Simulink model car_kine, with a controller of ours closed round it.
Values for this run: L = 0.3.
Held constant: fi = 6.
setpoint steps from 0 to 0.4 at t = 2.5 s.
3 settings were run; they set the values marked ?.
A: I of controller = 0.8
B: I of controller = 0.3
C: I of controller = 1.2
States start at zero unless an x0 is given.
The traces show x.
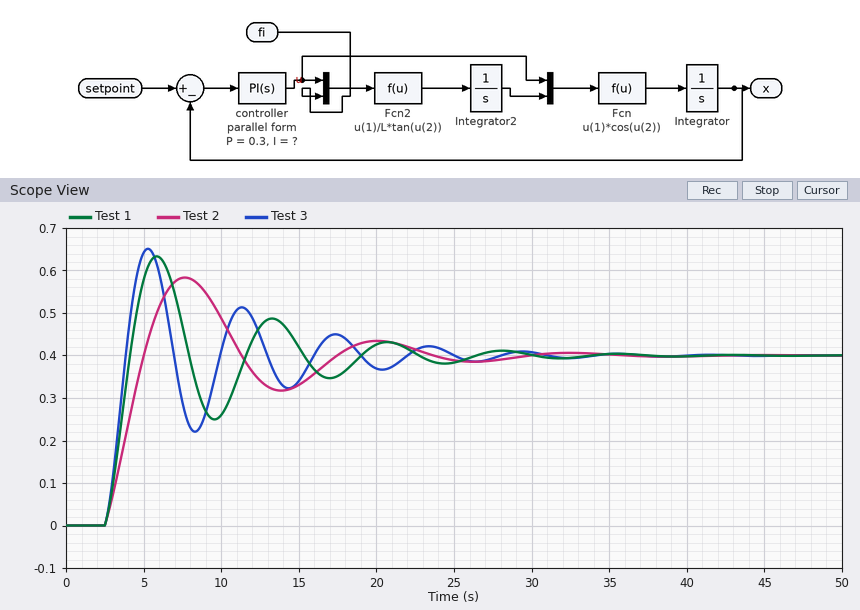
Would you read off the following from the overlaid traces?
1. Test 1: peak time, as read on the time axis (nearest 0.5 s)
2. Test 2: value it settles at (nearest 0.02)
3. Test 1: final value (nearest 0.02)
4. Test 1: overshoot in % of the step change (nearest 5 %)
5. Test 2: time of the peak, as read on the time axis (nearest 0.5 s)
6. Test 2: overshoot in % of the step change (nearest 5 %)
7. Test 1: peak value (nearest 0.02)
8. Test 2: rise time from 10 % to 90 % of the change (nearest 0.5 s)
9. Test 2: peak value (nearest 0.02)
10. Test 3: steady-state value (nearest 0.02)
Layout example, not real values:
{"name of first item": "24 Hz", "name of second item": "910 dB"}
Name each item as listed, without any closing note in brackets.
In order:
{"Test 1: peak time, as read on the time axis": "6.0 s", "Test 2: value it settles at": "0.40", "Test 1: final value": "0.40", "Test 1: overshoot in % of the step change": "60 %", "Test 2: time of the peak, as read on the time axis": "7.5 s", "Test 2: overshoot in % of the step change": "45 %", "Test 1: peak value": "0.64", "Test 2: rise time from 10 % to 90 % of the change": "2.0 s", "Test 2: peak value": "0.58", "Test 3: steady-state value": "0.40"}
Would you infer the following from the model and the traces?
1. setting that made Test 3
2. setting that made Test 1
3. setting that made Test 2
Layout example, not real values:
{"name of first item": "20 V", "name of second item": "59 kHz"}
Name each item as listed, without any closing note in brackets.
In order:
{"setting that made Test 3": "C", "setting that made Test 1": "A", "setting that made Test 2": "B"}
